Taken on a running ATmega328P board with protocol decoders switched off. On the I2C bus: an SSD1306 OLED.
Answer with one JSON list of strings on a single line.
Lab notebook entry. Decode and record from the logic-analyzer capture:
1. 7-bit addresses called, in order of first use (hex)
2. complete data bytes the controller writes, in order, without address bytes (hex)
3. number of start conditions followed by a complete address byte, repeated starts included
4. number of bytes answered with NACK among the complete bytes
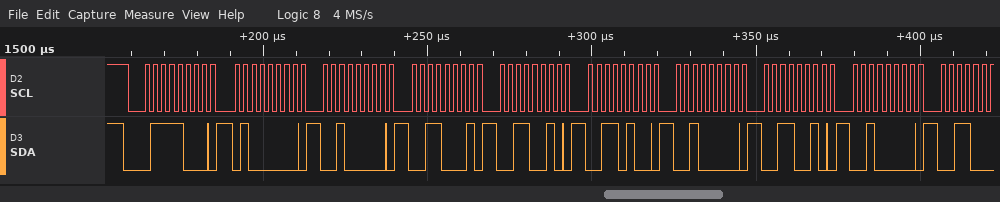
["0x3C", "40 20 31 32 34 20 32 20", "1", "0"]
